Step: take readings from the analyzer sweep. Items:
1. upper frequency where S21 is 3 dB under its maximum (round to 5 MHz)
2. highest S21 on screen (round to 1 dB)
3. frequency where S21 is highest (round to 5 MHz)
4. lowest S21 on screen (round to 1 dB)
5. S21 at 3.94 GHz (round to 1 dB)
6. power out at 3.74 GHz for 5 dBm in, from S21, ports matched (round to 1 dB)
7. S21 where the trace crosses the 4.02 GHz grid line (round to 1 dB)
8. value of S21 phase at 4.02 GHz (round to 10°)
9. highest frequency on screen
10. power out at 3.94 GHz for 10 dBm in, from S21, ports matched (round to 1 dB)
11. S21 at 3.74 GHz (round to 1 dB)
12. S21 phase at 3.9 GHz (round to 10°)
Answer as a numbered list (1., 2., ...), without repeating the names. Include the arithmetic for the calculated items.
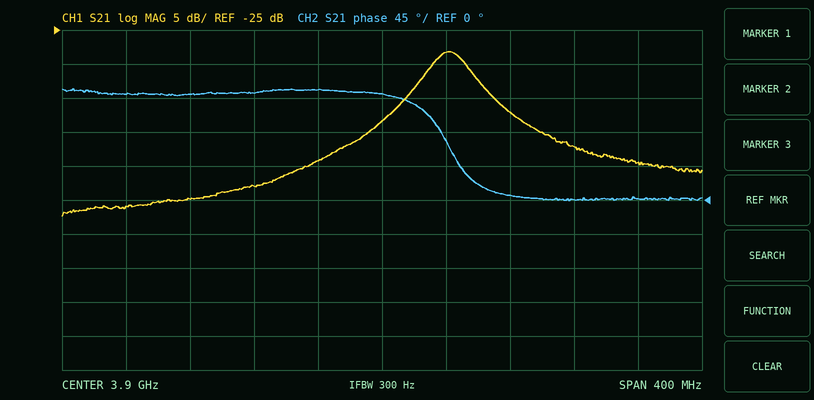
1. 3.955 GHz
2. -28 dB
3. 3.940 GHz
4. -52 dB
5. -28 dB
6. 5 dBm + (-51 dB) = -46 dBm
7. -42 dB
8. 0°
9. 4.1 GHz
10. 10 dBm + (-28 dB) = -18 dBm
11. -51 dB
12. 140°
